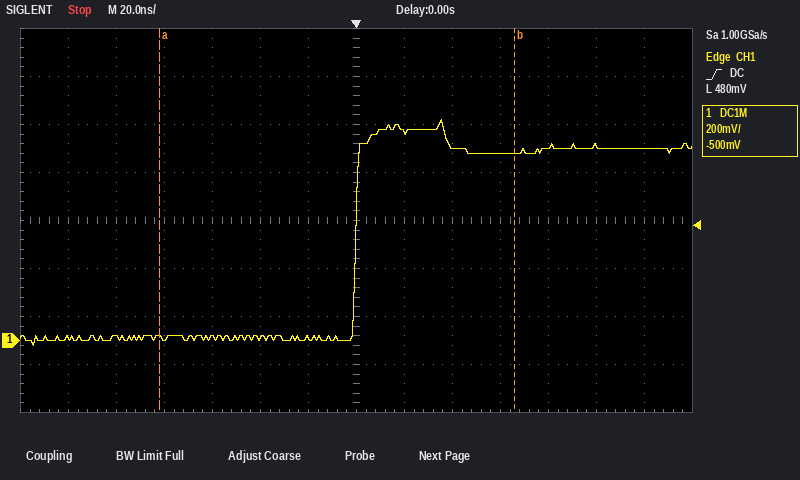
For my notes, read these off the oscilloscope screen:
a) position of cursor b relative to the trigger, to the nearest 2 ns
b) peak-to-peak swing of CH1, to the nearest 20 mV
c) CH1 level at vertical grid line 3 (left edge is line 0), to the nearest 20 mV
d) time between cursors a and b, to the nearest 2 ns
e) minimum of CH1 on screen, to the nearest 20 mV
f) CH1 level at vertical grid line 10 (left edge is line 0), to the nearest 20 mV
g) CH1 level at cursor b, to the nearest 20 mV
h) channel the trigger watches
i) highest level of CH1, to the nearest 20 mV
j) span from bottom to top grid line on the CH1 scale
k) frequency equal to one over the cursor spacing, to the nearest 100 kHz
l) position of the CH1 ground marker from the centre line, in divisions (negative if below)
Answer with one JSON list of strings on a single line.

["+66 ns", "940 mV", "0 mV", "148 ns", "-20 mV", "780 mV", "780 mV", "CH1", "920 mV", "1.6 V", "6.8 MHz", "-2.5 div"]
